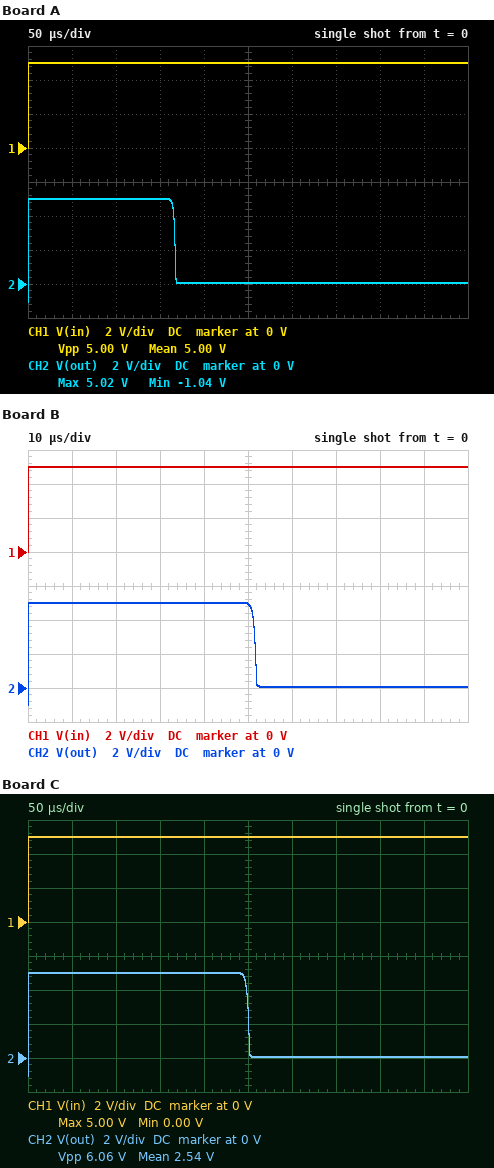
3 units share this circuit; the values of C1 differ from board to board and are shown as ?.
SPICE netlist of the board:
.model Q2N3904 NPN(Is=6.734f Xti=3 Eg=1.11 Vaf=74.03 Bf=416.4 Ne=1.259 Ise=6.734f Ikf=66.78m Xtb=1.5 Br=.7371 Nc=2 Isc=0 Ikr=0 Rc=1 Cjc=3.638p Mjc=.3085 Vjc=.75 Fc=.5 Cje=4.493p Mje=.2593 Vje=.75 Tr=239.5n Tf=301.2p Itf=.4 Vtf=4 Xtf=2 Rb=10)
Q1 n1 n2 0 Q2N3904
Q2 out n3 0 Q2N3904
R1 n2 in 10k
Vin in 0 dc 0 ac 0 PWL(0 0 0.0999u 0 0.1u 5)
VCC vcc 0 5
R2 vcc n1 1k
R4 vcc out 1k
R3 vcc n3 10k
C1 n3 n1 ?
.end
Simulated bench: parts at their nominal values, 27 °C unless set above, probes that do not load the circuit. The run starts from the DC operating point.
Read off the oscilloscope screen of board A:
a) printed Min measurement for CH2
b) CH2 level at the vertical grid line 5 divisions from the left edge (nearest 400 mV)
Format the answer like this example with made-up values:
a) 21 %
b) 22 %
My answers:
a) -1.04 V
b) 0 V
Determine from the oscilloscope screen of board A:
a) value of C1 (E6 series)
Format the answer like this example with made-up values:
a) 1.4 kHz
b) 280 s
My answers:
a) 22 nF
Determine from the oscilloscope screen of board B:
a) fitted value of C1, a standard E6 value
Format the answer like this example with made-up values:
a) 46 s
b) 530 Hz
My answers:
a) 6.8 nF
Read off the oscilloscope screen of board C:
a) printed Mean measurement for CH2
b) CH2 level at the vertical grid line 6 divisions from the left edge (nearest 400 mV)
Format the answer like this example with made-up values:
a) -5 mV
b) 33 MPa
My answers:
a) 2.54 V
b) 0 V
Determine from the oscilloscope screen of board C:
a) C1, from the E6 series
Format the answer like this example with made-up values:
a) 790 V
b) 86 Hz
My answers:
a) 33 nF
